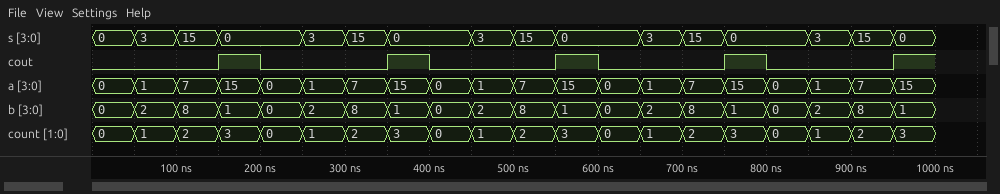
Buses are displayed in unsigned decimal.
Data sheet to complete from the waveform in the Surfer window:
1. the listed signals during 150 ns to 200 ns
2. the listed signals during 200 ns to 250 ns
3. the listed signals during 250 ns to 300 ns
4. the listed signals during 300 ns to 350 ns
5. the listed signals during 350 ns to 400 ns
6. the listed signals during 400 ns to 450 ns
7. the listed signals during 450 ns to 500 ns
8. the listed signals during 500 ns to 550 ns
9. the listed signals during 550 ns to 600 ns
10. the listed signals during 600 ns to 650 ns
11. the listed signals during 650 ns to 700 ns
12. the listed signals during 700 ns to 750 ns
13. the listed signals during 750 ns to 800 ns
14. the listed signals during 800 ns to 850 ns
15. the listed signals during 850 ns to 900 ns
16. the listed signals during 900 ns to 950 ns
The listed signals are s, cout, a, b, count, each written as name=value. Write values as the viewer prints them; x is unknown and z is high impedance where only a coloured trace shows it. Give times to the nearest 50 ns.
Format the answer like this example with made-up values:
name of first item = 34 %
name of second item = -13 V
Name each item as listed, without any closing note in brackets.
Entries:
the listed signals during 150 ns to 200 ns = s=0, cout=1, a=15, b=1, count=3
the listed signals during 200 ns to 250 ns = s=0, cout=0, a=0, b=0, count=0
the listed signals during 250 ns to 300 ns = s=3, cout=0, a=1, b=2, count=1
the listed signals during 300 ns to 350 ns = s=15, cout=0, a=7, b=8, count=2
the listed signals during 350 ns to 400 ns = s=0, cout=1, a=15, b=1, count=3
the listed signals during 400 ns to 450 ns = s=0, cout=0, a=0, b=0, count=0
the listed signals during 450 ns to 500 ns = s=3, cout=0, a=1, b=2, count=1
the listed signals during 500 ns to 550 ns = s=15, cout=0, a=7, b=8, count=2
the listed signals during 550 ns to 600 ns = s=0, cout=1, a=15, b=1, count=3
the listed signals during 600 ns to 650 ns = s=0, cout=0, a=0, b=0, count=0
the listed signals during 650 ns to 700 ns = s=3, cout=0, a=1, b=2, count=1
the listed signals during 700 ns to 750 ns = s=15, cout=0, a=7, b=8, count=2
the listed signals during 750 ns to 800 ns = s=0, cout=1, a=15, b=1, count=3
the listed signals during 800 ns to 850 ns = s=0, cout=0, a=0, b=0, count=0
the listed signals during 850 ns to 900 ns = s=3, cout=0, a=1, b=2, count=1
the listed signals during 900 ns to 950 ns = s=15, cout=0, a=7, b=8, count=2
